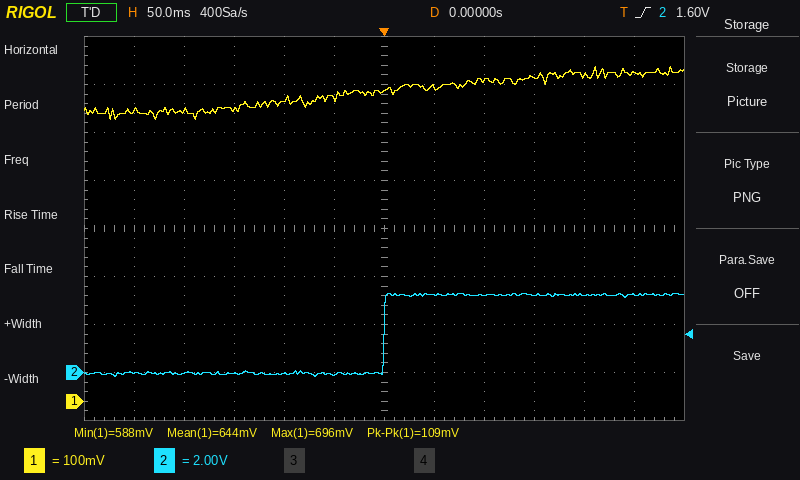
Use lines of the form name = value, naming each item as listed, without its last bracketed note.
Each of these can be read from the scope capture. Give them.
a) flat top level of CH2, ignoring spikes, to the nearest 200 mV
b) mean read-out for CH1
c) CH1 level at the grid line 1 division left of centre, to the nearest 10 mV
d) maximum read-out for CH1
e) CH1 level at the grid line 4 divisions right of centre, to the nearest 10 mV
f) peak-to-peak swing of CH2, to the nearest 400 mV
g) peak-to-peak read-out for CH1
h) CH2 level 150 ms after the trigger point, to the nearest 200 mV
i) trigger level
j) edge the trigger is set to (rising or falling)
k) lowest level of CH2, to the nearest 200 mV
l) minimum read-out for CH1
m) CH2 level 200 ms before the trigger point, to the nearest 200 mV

flat top level of CH2, ignoring spikes, to the nearest 200 mV = 3.2 V
mean read-out for CH1 = 644 mV
CH1 level at the grid line 1 division left of centre, to the nearest 10 mV = 630 mV
maximum read-out for CH1 = 696 mV
CH1 level at the grid line 4 divisions right of centre, to the nearest 10 mV = 680 mV
peak-to-peak swing of CH2, to the nearest 400 mV = 3.6 V
peak-to-peak read-out for CH1 = 109 mV
CH2 level 150 ms after the trigger point, to the nearest 200 mV = 3.2 V
trigger level = 1.60 V
edge the trigger is set to = rising
lowest level of CH2, to the nearest 200 mV = -200 mV
minimum read-out for CH1 = 588 mV
CH2 level 200 ms before the trigger point, to the nearest 200 mV = 0.0 V
